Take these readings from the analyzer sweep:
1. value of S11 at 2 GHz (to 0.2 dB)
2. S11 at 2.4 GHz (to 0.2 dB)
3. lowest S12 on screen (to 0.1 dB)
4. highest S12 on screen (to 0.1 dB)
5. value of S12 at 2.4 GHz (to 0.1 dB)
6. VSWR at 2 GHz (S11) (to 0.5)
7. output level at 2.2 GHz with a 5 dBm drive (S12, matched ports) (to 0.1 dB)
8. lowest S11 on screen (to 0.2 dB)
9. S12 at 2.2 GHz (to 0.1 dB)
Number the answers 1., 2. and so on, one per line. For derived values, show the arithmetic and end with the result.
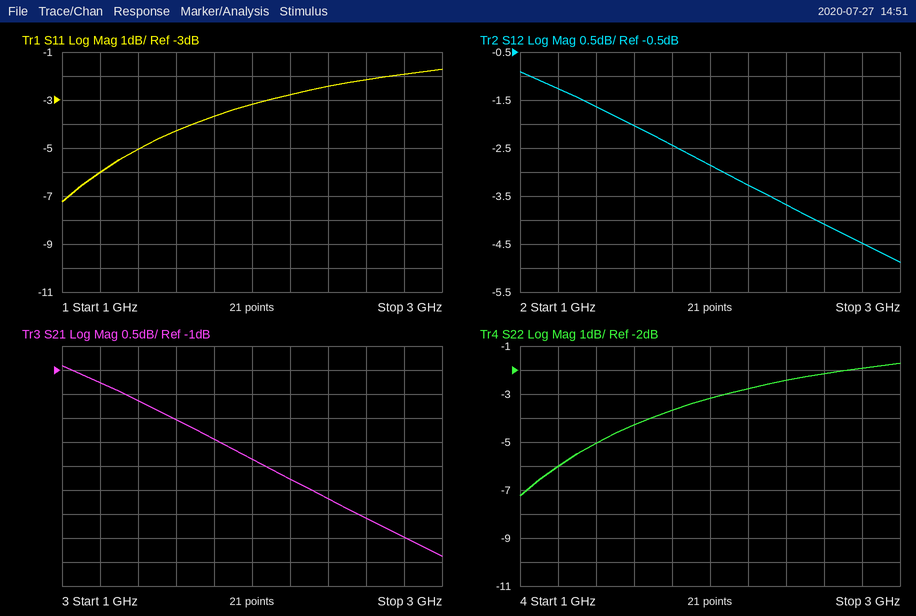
1. -3.2 dB
2. -2.4 dB
3. -4.9 dB
4. -0.9 dB
5. -3.7 dB
6. |Γ| = 10^(-3.2/20) = 0.6918; VSWR = (1 + 0.6918)/(1 − 0.6918) ≈ 5.5
7. 5 dBm + (-3.3 dB) = 1.7 dBm
8. -7.2 dB
9. -3.3 dB
